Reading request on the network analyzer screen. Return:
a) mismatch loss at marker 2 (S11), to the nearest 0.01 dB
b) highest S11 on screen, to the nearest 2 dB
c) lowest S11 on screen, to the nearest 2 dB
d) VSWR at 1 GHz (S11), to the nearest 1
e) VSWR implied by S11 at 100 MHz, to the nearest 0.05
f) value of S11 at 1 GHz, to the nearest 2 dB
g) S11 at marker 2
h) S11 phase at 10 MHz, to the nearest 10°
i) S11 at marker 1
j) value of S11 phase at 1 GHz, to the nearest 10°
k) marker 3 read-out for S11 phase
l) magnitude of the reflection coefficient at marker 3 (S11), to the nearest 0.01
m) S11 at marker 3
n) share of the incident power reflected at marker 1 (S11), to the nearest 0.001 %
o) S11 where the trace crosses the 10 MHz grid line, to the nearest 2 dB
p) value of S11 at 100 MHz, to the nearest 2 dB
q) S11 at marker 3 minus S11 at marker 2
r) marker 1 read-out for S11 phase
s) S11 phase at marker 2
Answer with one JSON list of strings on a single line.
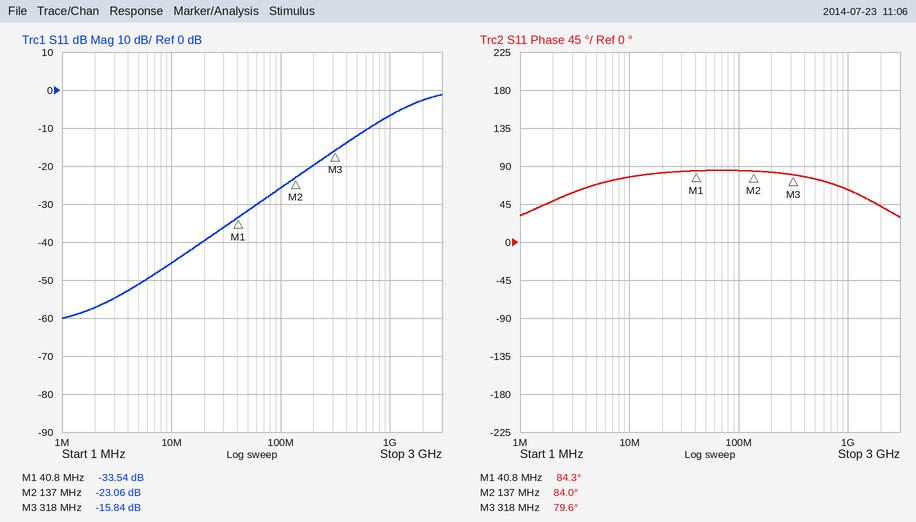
["0.02 dB", "-2 dB", "-60 dB", "3", "1.10", "-6 dB", "-23.06 dB", "80°", "-33.54 dB", "60°", "79.6°", "0.16", "-15.84 dB", "0.044 %", "-46 dB", "-26 dB", "7.22 dB", "84.3°", "84.0°"]
